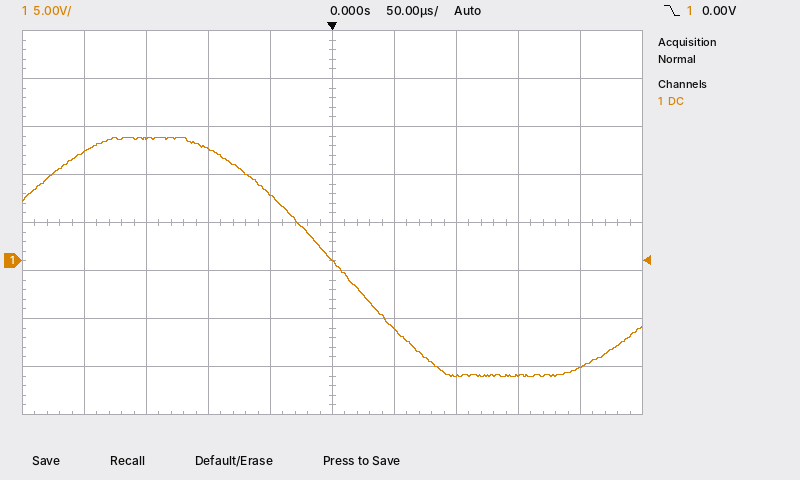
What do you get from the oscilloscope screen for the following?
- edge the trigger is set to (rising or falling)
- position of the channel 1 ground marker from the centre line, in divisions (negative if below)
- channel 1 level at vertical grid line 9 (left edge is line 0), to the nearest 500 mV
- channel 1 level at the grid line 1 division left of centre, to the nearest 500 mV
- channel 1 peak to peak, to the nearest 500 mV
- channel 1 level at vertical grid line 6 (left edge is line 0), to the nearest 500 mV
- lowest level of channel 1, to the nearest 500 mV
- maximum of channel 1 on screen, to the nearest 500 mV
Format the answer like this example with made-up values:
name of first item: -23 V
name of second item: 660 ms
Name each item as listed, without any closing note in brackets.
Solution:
edge the trigger is set to: falling
position of the channel 1 ground marker from the centre line, in divisions: -0.8 div
channel 1 level at vertical grid line 9 (left edge is line 0), to the nearest 500 mV: -11.0 V
channel 1 level at the grid line 1 division left of centre, to the nearest 500 mV: 7.0 V
channel 1 peak to peak, to the nearest 500 mV: 25.0 V
channel 1 level at vertical grid line 6 (left edge is line 0), to the nearest 500 mV: -7.0 V
lowest level of channel 1, to the nearest 500 mV: -12.0 V
maximum of channel 1 on screen, to the nearest 500 mV: 13.0 V
